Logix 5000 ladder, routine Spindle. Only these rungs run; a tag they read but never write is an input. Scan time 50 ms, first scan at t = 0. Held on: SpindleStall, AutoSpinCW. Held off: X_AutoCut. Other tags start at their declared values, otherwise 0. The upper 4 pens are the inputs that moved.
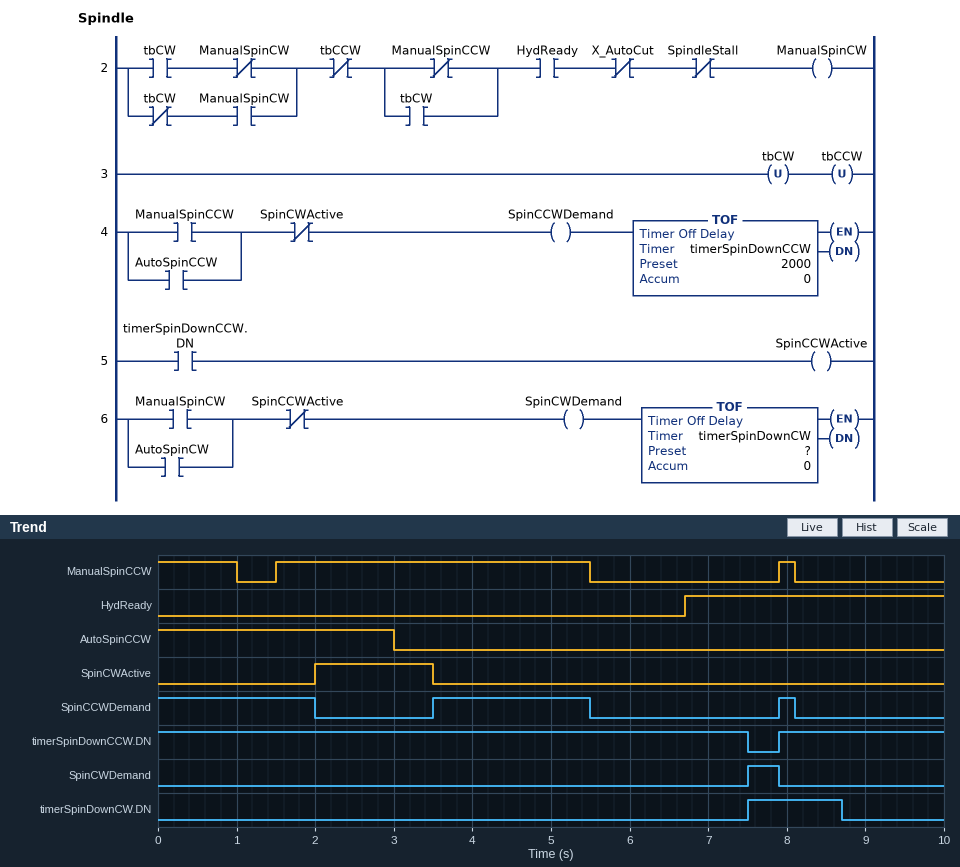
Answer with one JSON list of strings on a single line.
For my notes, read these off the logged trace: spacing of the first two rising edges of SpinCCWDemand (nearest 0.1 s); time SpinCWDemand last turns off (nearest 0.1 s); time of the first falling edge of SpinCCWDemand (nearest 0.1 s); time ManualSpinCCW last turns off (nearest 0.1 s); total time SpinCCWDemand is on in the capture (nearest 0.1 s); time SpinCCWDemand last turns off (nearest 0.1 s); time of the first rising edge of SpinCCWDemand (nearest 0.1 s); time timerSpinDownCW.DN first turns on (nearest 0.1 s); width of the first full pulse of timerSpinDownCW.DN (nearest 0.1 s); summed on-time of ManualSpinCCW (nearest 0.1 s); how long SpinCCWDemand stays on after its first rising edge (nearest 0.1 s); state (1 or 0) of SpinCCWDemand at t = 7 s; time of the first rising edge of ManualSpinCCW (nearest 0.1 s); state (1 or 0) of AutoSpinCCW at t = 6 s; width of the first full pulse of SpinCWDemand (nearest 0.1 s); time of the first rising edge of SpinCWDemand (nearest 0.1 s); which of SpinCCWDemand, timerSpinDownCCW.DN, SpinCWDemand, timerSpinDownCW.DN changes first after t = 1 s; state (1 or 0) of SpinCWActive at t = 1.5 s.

["4.4 s", "7.9 s", "2.0 s", "8.1 s", "4.2 s", "8.1 s", "3.5 s", "7.5 s", "1.2 s", "5.2 s", "2.0 s", "0", "1.5 s", "0", "0.4 s", "7.5 s", "SpinCCWDemand", "0"]
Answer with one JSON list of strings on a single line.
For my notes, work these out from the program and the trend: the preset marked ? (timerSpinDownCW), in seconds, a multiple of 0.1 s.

["0.8 s"]
